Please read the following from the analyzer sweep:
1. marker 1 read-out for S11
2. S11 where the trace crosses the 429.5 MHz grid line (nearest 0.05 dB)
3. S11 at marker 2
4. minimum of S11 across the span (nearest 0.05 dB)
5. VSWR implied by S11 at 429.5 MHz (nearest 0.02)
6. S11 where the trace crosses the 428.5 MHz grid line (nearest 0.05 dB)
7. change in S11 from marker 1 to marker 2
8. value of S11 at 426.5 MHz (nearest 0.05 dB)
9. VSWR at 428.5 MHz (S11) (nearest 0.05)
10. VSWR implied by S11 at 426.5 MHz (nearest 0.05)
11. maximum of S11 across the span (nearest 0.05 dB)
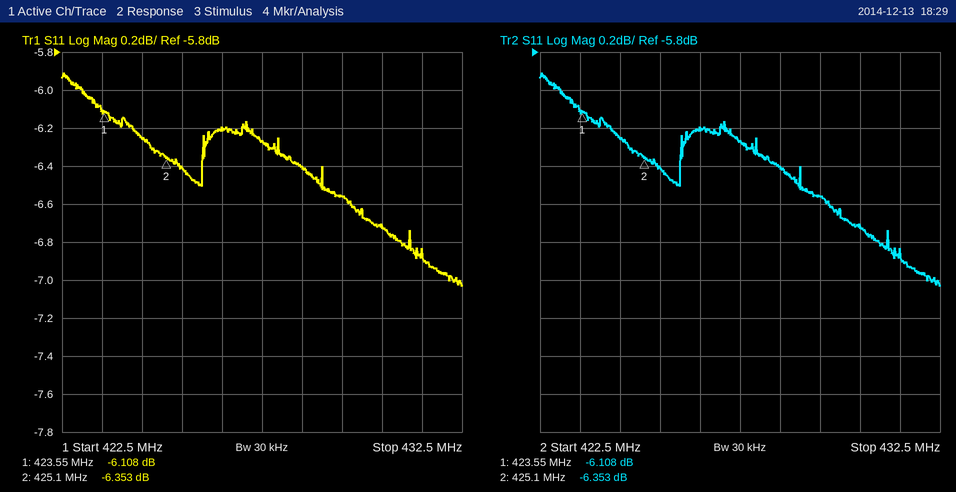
-6.108 dB
-6.55 dB
-6.353 dB
-7.05 dB
2.78
-6.40 dB
-0.245 dB
-6.20 dB
2.85
2.90
-5.90 dB
